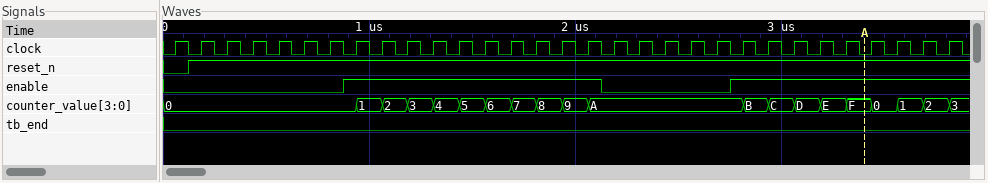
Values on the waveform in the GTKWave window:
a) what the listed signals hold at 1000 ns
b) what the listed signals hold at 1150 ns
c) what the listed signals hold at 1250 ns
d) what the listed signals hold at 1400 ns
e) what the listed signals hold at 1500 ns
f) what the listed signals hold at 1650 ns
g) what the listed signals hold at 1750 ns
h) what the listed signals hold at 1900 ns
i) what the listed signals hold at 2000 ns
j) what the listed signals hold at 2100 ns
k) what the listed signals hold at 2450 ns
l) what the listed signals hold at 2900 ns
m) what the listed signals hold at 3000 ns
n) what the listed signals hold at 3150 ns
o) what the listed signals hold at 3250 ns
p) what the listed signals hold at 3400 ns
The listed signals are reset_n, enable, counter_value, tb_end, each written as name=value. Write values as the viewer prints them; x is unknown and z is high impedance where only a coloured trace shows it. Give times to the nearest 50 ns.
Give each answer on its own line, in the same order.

reset_n=1, enable=1, counter_value=1, tb_end=0
reset_n=1, enable=1, counter_value=2, tb_end=0
reset_n=1, enable=1, counter_value=3, tb_end=0
reset_n=1, enable=1, counter_value=4, tb_end=0
reset_n=1, enable=1, counter_value=5, tb_end=0
reset_n=1, enable=1, counter_value=6, tb_end=0
reset_n=1, enable=1, counter_value=7, tb_end=0
reset_n=1, enable=1, counter_value=8, tb_end=0
reset_n=1, enable=1, counter_value=9, tb_end=0
reset_n=1, enable=1, counter_value=A, tb_end=0
reset_n=1, enable=0, counter_value=A, tb_end=0
reset_n=1, enable=1, counter_value=B, tb_end=0
reset_n=1, enable=1, counter_value=C, tb_end=0
reset_n=1, enable=1, counter_value=D, tb_end=0
reset_n=1, enable=1, counter_value=E, tb_end=0
reset_n=1, enable=1, counter_value=F, tb_end=0
